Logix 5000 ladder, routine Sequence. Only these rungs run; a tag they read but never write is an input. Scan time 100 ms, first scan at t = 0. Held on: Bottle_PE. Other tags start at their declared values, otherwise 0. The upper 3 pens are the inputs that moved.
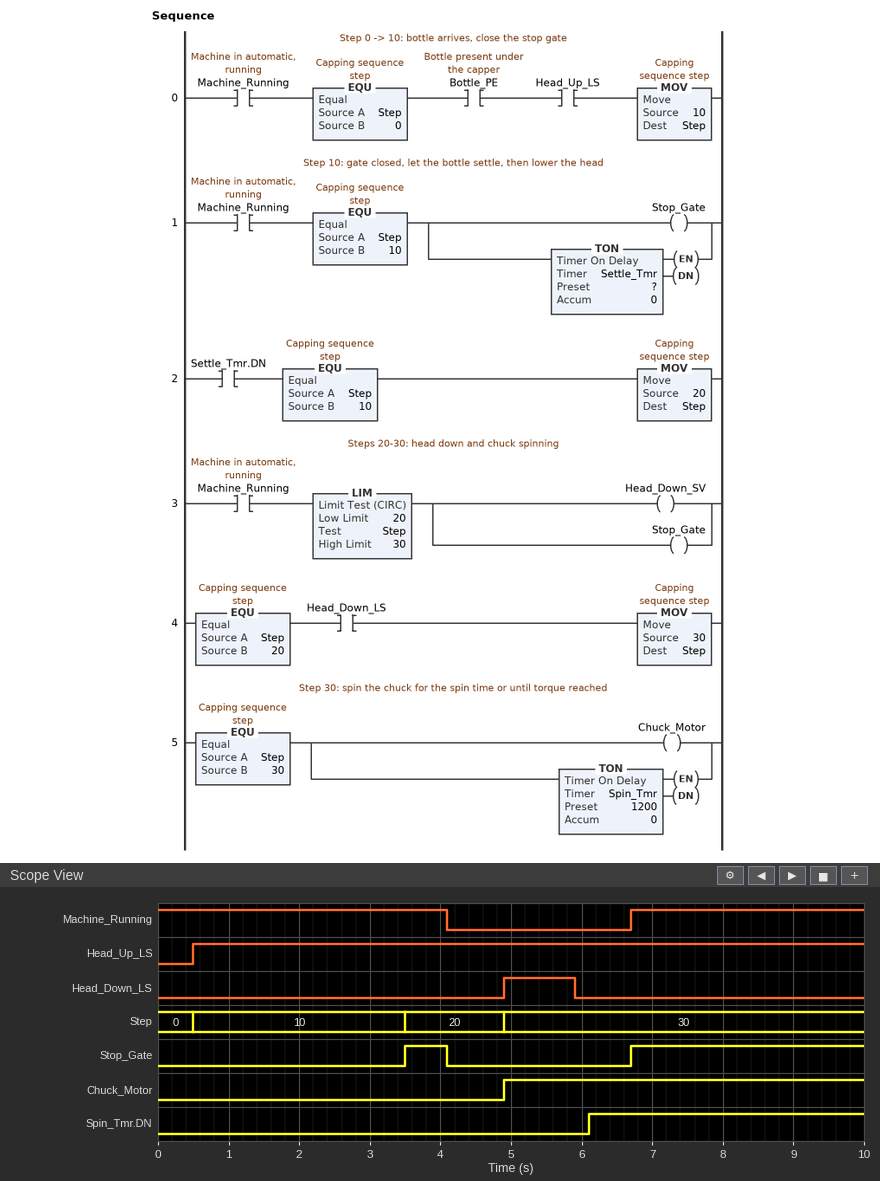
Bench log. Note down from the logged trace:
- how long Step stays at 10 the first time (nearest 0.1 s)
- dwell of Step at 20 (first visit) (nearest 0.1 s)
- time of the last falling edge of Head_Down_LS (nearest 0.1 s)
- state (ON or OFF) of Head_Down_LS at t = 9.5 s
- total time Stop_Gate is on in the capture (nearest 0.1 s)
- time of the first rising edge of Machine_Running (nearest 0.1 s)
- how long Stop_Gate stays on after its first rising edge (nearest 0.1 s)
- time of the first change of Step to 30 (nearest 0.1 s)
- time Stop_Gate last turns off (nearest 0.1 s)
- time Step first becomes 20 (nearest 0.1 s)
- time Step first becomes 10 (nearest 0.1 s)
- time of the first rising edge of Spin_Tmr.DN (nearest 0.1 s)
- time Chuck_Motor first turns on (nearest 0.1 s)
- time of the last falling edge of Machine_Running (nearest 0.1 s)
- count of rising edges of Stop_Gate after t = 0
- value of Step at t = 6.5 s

3.0 s
1.4 s
5.9 s
OFF
3.9 s
6.7 s
0.6 s
4.9 s
4.1 s
3.5 s
0.5 s
6.1 s
4.9 s
4.1 s
2
30
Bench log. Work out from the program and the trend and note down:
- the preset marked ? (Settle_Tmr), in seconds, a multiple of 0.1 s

3.0 s
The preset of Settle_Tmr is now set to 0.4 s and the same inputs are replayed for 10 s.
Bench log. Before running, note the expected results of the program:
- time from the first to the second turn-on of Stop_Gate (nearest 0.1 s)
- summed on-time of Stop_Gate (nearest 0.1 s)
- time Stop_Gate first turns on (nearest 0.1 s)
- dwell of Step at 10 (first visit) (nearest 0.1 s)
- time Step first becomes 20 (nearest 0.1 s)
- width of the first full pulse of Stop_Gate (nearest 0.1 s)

5.8 s
6.5 s
0.9 s
0.4 s
0.9 s
3.2 s
